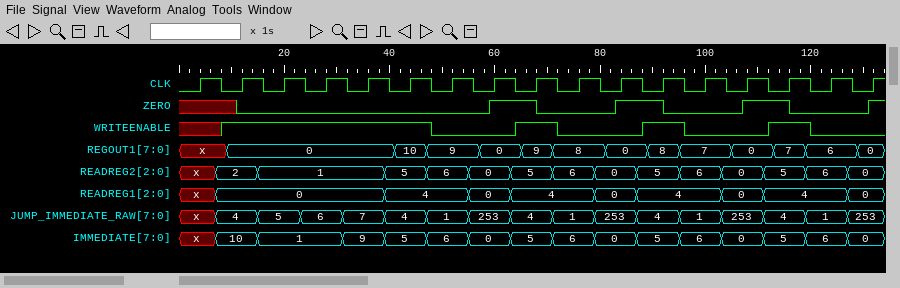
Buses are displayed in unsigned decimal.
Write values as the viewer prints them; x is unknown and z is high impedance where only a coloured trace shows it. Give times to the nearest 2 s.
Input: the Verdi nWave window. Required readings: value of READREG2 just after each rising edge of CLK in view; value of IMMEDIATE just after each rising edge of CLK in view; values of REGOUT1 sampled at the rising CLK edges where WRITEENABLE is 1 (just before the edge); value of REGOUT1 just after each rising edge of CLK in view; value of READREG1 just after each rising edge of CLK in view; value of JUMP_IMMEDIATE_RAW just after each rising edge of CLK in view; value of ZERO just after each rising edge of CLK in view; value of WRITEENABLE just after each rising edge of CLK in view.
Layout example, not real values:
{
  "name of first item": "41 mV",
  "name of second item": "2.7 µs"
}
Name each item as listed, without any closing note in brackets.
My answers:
{
  "value of READREG2 just after each rising edge of CLK in view": "x, 2, 1, 1, 1, 5, 6, 0, 5, 6, 0, 5, 6, 0, 5, 6, 0",
  "value of IMMEDIATE just after each rising edge of CLK in view": "x, 10, 1, 1, 9, 5, 6, 0, 5, 6, 0, 5, 6, 0, 5, 6, 0",
  "values of REGOUT1 sampled at the rising CLK edges where WRITEENABLE is 1": "0, 0, 0, 0, 10, 9, 8, 7",
  "value of REGOUT1 just after each rising edge of CLK in view": "x, 0, 0, 0, 0, 10, 9, 0, 9, 8, 0, 8, 7, 0, 7, 6, 0",
  "value of READREG1 just after each rising edge of CLK in view": "x, 0, 0, 0, 0, 4, 4, 0, 4, 4, 0, 4, 4, 0, 4, 4, 0",
  "value of JUMP_IMMEDIATE_RAW just after each rising edge of CLK in view": "x, 4, 5, 6, 7, 4, 1, 253, 4, 1, 253, 4, 1, 253, 4, 1, 253",
  "value of ZERO just after each rising edge of CLK in view": "x 0 0 0 0 0 0 1 0 0 1 0 0 1 0 0 1",
  "value of WRITEENABLE just after each rising edge of CLK in view": "x 1 1 1 1 1 0 0 1 0 0 1 0 0 1 0 0"
}
